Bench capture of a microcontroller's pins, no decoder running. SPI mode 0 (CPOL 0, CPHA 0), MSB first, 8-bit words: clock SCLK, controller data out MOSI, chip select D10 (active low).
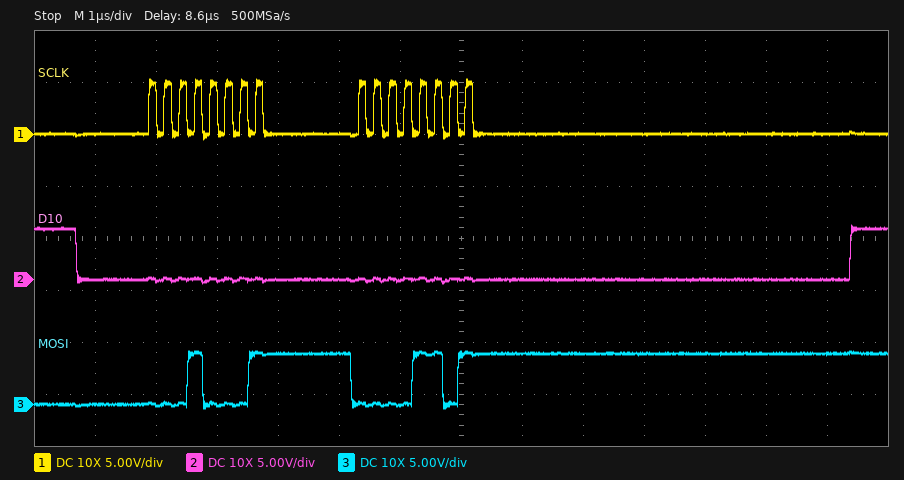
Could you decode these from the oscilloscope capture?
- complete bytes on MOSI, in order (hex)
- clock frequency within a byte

11 0D
4 MHz
